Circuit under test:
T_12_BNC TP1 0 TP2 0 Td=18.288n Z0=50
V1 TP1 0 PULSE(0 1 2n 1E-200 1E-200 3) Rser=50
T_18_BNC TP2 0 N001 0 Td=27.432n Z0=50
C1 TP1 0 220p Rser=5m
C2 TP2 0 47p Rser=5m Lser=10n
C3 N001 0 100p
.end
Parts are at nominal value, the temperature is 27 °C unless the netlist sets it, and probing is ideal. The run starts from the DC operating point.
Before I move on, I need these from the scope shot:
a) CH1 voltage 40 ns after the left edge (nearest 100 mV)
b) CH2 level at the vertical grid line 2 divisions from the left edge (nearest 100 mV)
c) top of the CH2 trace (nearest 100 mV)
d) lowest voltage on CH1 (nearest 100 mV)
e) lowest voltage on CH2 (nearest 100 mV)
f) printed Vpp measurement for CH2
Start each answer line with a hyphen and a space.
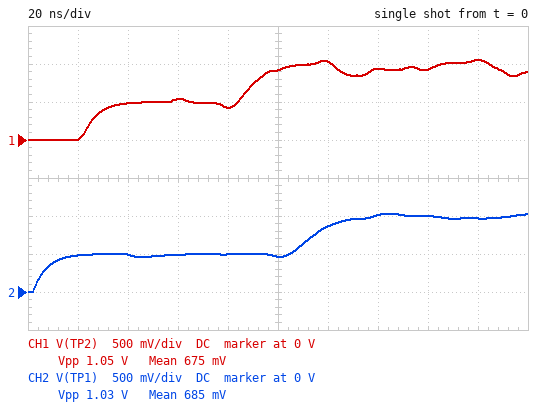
- 500 mV
- 500 mV
- 1.0 V
- 0 V
- 0 V
- 1.03 V
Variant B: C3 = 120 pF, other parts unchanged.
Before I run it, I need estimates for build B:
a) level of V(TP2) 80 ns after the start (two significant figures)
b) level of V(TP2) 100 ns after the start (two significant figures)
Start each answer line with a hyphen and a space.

- 410 mV
- 890 mV
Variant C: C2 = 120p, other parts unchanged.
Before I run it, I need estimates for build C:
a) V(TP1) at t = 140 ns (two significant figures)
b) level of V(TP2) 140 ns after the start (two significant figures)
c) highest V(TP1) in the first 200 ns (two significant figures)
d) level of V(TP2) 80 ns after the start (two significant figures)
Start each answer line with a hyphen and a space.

- 980 mV
- 880 mV
- 1.1 V
- 450 mV
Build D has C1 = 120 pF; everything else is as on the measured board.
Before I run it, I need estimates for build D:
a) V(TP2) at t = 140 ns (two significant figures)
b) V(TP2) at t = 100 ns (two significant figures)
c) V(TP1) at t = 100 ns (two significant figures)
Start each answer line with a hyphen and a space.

- 1.0 V
- 950 mV
- 430 mV
